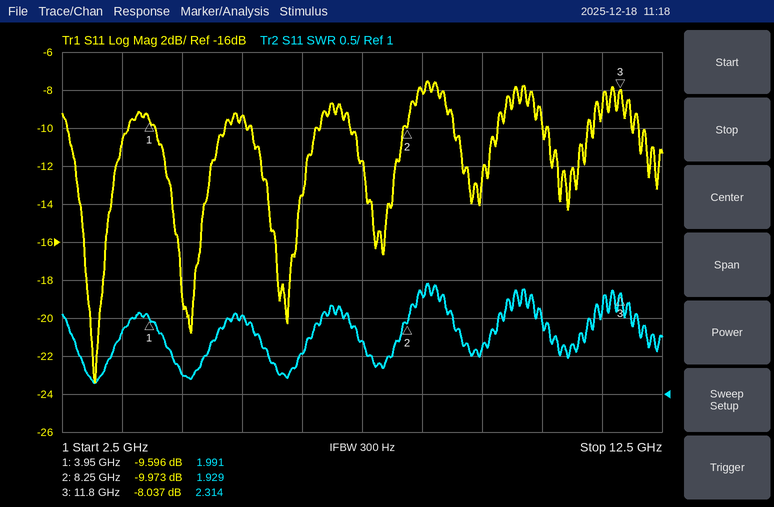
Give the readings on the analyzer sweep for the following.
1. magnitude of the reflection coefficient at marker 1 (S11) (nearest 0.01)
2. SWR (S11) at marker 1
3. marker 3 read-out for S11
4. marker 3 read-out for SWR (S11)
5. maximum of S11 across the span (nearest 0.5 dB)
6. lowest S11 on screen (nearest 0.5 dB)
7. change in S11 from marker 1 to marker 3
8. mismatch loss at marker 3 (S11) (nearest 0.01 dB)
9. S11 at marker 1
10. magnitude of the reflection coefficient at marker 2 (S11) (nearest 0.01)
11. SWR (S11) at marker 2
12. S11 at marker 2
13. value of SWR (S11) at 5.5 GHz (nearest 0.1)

0.33
1.991
-8.037 dB
2.314
-7.5 dB
-23.5 dB
1.559 dB
0.74 dB
-9.596 dB
0.32
1.929
-9.973 dB
2.0
